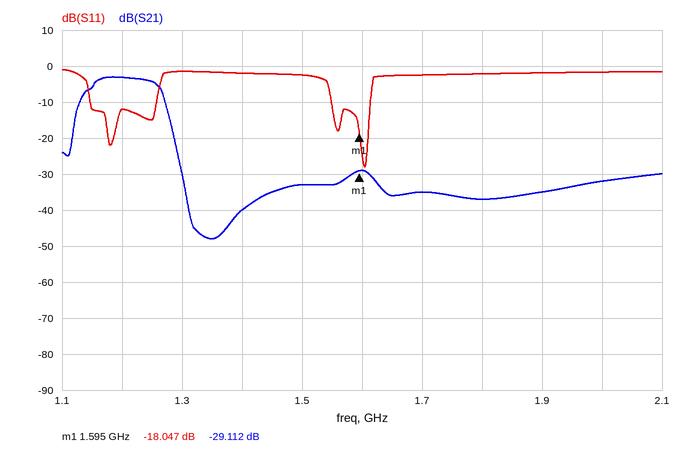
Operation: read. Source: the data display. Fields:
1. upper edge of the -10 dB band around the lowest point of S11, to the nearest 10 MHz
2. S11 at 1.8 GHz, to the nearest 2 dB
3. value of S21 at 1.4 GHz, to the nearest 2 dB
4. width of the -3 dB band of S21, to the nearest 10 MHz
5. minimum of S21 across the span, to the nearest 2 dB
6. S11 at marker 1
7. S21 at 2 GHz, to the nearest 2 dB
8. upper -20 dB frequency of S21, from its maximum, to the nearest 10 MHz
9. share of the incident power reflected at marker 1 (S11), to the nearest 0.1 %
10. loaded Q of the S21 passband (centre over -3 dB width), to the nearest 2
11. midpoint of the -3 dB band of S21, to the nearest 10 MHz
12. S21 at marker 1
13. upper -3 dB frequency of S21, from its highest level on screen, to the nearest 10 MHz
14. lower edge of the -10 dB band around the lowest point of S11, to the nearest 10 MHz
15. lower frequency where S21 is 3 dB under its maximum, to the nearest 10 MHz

1.61 GHz
-2 dB
-40 dB
110 MHz
-48 dB
-18.047 dB
-32 dB
1.29 GHz
1.6 %
10
1.21 GHz
-29.112 dB
1.26 GHz
1.55 GHz
1.15 GHz
